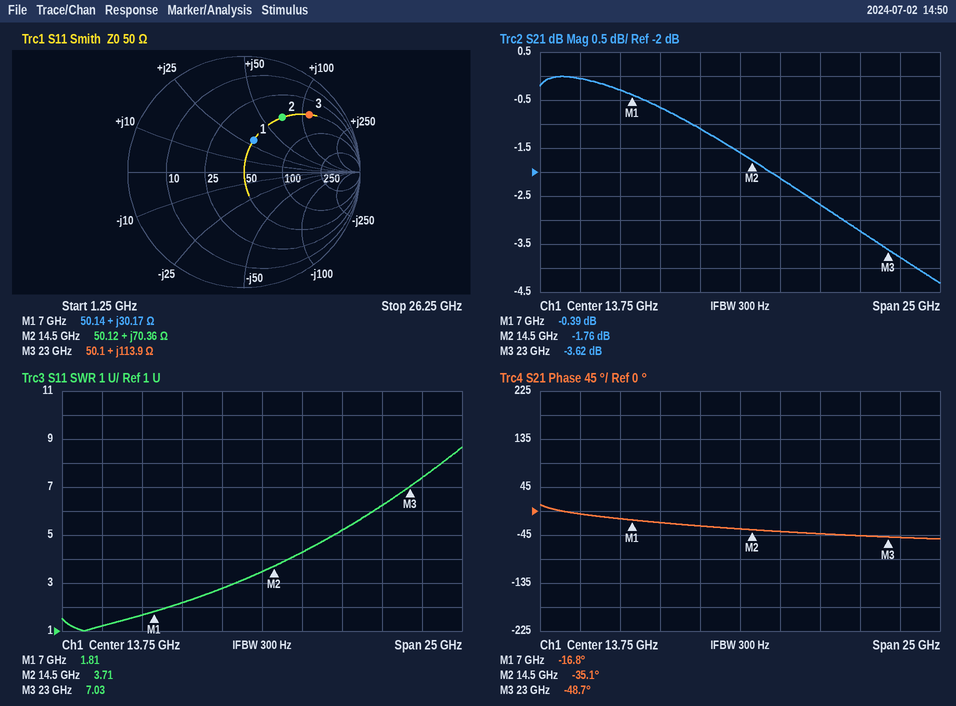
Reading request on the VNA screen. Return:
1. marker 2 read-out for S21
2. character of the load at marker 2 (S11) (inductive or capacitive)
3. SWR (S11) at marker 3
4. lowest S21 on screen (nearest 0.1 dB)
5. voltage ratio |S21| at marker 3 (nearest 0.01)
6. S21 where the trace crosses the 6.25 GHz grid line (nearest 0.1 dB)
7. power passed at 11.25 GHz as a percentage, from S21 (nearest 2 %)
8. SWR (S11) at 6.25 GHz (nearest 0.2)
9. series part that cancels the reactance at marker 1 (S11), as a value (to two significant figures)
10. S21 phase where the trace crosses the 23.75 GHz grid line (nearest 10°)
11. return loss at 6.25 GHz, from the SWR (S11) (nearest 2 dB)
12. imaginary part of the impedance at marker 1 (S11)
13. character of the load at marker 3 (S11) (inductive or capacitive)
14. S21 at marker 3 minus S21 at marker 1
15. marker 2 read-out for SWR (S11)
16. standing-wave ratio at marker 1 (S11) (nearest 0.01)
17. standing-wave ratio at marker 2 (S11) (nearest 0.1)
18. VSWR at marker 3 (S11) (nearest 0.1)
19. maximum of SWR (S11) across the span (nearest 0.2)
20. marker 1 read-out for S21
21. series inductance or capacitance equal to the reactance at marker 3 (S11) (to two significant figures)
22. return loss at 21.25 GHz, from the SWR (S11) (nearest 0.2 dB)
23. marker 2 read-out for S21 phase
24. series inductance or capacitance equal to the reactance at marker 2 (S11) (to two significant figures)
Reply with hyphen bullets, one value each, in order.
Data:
- -1.76 dB
- inductive
- 7.03
- -4.3 dB
- 0.66
- -0.3 dB
- 78 %
- 1.6
- 750 fF
- -50°
- 12 dB
- +30.17 Ω
- inductive
- -3.23 dB
- 3.71
- 1.81
- 3.7
- 7.0
- 8.6
- -0.39 dB
- 790 pH
- 2.8 dB
- -35.1°
- 770 pH
